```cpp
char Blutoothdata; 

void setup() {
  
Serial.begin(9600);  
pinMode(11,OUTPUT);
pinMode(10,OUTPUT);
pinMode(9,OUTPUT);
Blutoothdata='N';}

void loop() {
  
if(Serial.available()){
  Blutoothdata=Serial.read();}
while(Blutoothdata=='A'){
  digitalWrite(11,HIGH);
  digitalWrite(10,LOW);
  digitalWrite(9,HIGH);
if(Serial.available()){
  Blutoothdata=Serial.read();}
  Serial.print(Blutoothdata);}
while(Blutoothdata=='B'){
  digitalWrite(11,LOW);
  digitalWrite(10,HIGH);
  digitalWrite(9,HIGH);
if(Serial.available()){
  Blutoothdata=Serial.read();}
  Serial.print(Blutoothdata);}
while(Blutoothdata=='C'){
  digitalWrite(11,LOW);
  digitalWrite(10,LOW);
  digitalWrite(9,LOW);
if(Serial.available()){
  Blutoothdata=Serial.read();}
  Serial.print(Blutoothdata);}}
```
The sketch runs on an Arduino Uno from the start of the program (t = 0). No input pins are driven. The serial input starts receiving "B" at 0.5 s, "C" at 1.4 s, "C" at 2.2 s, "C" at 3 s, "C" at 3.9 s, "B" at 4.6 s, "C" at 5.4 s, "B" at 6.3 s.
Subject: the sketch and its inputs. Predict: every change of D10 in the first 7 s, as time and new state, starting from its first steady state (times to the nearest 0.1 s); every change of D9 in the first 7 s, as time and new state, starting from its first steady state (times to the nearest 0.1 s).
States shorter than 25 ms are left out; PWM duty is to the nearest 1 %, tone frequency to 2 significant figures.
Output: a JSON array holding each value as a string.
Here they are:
["0 s low; 0.5 s high; 1.4 s low; 4.6 s high; 5.4 s low; 6.3 s high", "0 s low; 0.5 s high; 1.4 s low; 4.6 s high; 5.4 s low; 6.3 s high"]
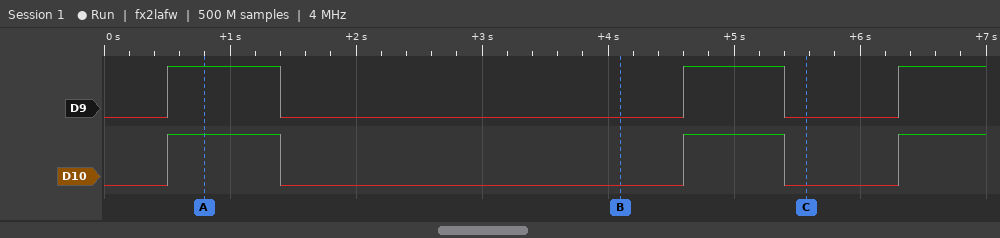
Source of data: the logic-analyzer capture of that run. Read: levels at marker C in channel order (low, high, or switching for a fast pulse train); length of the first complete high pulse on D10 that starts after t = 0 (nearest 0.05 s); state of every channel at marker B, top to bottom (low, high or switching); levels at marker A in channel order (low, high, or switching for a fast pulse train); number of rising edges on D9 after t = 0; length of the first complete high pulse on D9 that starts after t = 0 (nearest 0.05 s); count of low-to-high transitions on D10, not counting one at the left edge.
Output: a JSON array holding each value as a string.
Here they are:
["D9 low, D10 low", "0.90 s", "D9 low, D10 low", "D9 high, D10 high", "3", "0.90 s", "3"]
